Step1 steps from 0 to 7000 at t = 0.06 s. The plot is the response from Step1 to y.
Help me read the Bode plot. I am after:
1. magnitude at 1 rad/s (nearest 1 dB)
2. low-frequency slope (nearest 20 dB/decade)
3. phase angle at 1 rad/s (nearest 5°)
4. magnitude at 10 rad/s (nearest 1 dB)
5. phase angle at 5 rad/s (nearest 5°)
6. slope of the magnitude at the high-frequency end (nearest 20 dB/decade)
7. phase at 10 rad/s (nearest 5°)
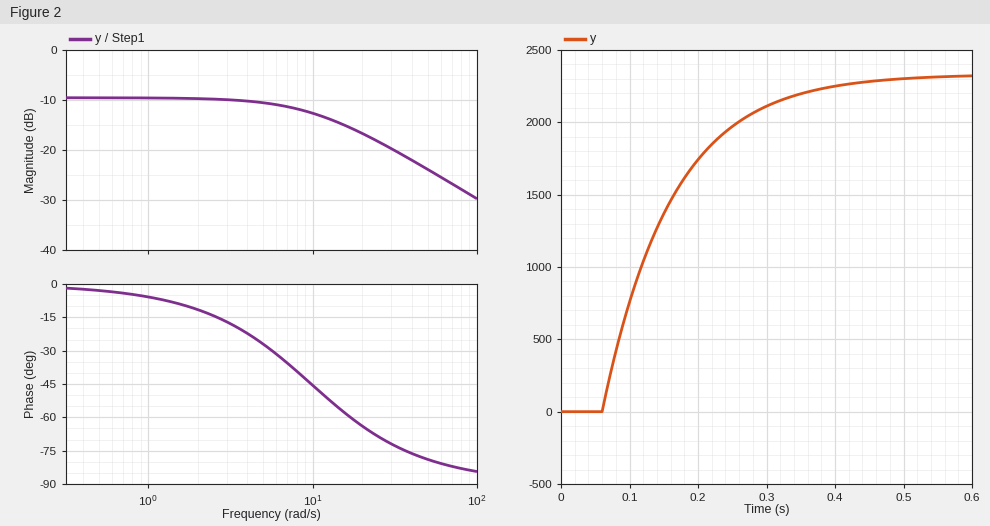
-10 dB
0 dB/decade
-5°
-13 dB
-25°
-20 dB/decade
-45°
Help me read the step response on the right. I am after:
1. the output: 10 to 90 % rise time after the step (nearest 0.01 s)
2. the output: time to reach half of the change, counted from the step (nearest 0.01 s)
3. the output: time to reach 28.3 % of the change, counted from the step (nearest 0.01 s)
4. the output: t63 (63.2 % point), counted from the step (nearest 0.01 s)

0.22 s
0.07 s
0.03 s
0.10 s
